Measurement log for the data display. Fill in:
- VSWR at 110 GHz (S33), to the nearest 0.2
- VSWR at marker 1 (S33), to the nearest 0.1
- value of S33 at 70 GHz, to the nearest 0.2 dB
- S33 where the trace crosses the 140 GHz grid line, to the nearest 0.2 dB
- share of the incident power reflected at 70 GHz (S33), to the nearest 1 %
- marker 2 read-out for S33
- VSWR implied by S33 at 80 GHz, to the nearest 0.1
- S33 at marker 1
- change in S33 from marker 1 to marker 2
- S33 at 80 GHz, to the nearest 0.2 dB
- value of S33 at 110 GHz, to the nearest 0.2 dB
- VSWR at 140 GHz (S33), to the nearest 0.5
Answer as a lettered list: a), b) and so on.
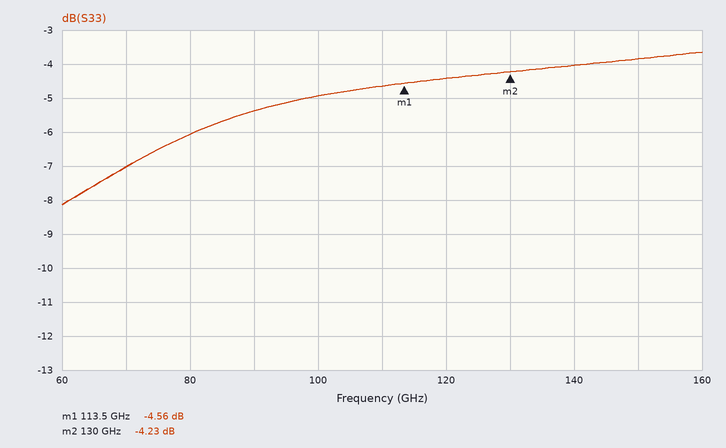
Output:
a) 3.8
b) 3.9
c) -7.0 dB
d) -4.0 dB
e) 20 %
f) -4.23 dB
g) 3.0
h) -4.56 dB
i) 0.33 dB
j) -6.0 dB
k) -4.6 dB
l) 4.5
